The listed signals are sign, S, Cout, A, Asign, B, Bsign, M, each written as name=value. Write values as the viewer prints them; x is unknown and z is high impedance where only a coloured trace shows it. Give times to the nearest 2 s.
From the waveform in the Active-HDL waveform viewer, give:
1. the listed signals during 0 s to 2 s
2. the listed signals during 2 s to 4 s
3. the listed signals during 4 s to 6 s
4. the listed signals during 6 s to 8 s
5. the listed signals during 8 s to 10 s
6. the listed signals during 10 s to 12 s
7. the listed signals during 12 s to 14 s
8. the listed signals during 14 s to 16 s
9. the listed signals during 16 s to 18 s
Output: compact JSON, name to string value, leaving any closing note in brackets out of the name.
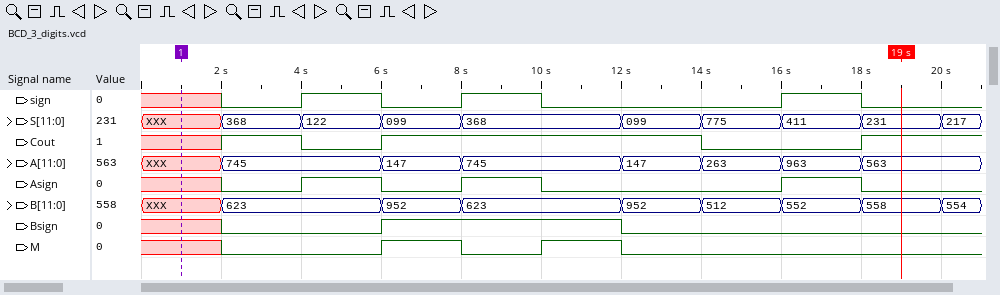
{"the listed signals during 0 s to 2 s": "sign=x, S=XXX, Cout=x, A=XXX, Asign=x, B=XXX, Bsign=x, M=x", "the listed signals during 2 s to 4 s": "sign=0, S=368, Cout=1, A=745, Asign=0, B=623, Bsign=0, M=0", "the listed signals during 4 s to 6 s": "sign=1, S=122, Cout=0, A=745, Asign=1, B=623, Bsign=0, M=0", "the listed signals during 6 s to 8 s": "sign=0, S=099, Cout=1, A=147, Asign=0, B=952, Bsign=1, M=1", "the listed signals during 8 s to 10 s": "sign=1, S=368, Cout=1, A=745, Asign=1, B=623, Bsign=1, M=0", "the listed signals during 10 s to 12 s": "sign=0, S=368, Cout=1, A=745, Asign=0, B=623, Bsign=1, M=1", "the listed signals during 12 s to 14 s": "sign=0, S=099, Cout=1, A=147, Asign=0, B=952, Bsign=0, M=0", "the listed signals during 14 s to 16 s": "sign=0, S=775, Cout=0, A=263, Asign=0, B=512, Bsign=0, M=0", "the listed signals during 16 s to 18 s": "sign=1, S=411, Cout=0, A=963, Asign=1, B=552, Bsign=0, M=0"}
